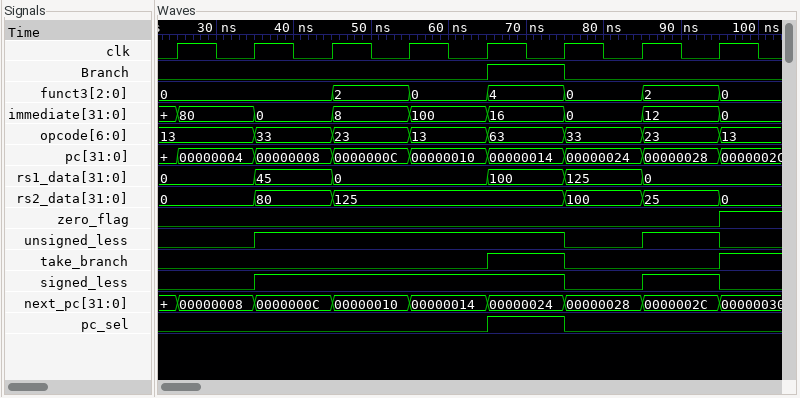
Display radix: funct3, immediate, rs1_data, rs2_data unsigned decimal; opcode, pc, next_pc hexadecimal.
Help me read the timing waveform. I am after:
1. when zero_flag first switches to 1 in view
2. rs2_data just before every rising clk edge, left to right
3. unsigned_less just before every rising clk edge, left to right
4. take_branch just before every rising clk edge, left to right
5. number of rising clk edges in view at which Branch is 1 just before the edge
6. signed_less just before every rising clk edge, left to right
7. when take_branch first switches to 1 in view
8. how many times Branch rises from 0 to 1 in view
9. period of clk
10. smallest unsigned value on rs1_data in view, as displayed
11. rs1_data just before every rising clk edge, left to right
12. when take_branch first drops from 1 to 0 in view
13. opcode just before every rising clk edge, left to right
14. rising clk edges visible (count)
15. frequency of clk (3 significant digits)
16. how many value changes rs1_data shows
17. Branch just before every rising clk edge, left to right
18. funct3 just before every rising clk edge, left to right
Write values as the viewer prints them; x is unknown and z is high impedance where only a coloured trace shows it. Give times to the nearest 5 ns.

95 ns
0, 0, 80, 125, 125, 125, 100, 25
0 0 1 1 1 1 0 1
0 0 0 0 0 1 0 0
1
0 0 1 1 1 1 0 1
65 ns
1
10 ns
0
0, 0, 45, 0, 0, 100, 125, 0
75 ns
13, 13, 33, 23, 13, 63, 33, 23
8
100 MHz
5
0 0 0 0 0 1 0 0
0, 0, 0, 2, 0, 4, 0, 2
